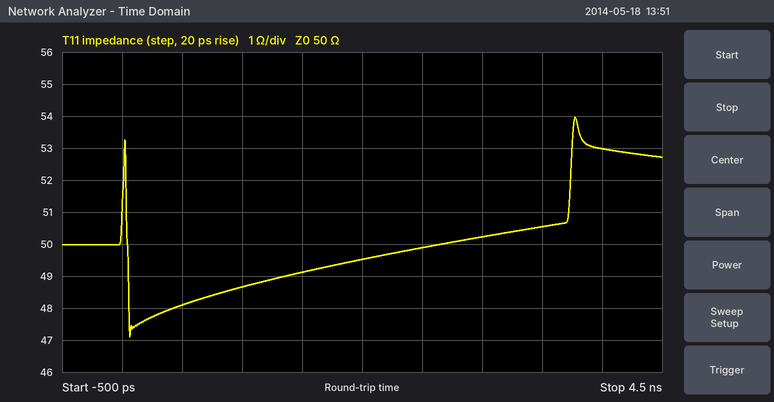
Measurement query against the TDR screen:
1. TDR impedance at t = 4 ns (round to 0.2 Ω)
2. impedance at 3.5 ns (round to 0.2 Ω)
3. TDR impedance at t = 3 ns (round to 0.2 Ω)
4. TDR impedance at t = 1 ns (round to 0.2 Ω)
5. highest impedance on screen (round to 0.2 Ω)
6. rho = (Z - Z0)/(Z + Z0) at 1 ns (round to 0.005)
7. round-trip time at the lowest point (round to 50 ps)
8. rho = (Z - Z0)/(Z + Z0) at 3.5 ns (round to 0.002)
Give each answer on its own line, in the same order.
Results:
53.0 Ω
50.6 Ω
50.2 Ω
48.6 Ω
54.0 Ω
-0.015
50 ps
+0.006
